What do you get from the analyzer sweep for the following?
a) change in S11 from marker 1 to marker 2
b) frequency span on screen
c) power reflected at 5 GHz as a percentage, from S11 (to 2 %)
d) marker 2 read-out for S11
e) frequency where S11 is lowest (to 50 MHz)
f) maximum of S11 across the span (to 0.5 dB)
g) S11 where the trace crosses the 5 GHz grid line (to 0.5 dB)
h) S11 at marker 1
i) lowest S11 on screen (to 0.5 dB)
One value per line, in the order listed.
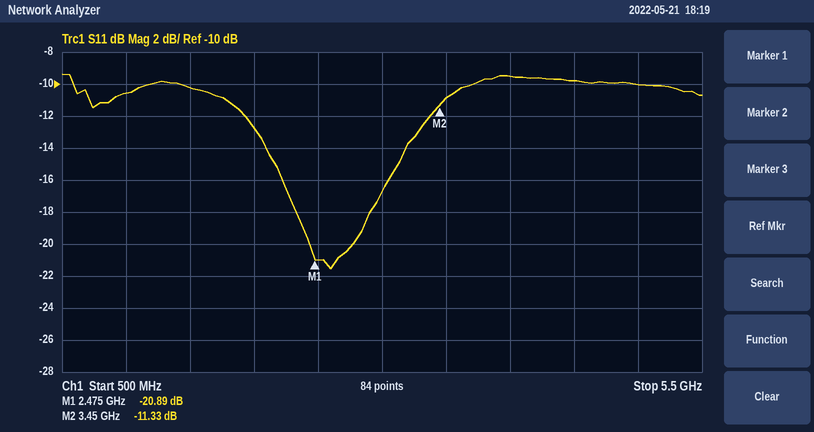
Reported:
9.56 dB
5 GHz
10 %
-11.33 dB
2.60 GHz
-9.5 dB
-10.0 dB
-20.89 dB
-21.5 dB
